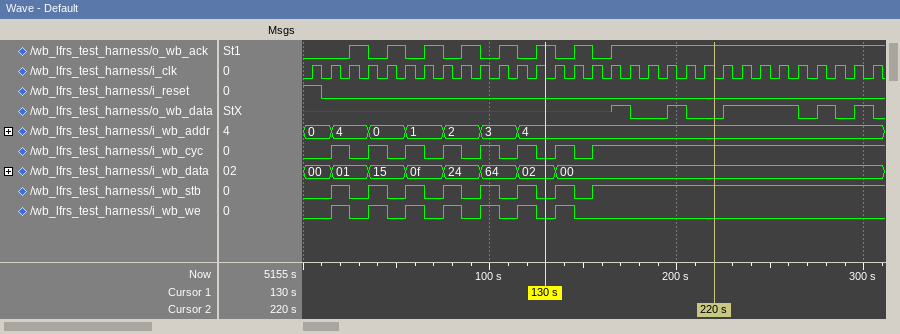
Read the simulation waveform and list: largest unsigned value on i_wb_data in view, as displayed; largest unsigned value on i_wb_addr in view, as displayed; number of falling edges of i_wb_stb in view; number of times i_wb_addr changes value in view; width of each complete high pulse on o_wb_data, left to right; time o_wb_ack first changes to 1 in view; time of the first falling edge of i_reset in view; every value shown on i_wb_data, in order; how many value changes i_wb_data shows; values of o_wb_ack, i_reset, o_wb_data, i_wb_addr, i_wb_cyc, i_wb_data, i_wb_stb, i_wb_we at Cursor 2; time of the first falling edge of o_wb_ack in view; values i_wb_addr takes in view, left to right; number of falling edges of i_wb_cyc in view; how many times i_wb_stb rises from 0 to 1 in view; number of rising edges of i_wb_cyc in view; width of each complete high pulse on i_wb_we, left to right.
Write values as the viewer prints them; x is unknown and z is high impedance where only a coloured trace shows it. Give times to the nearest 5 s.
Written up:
64
4
7
6
10 s, 40 s, 10 s, 10 s
25 s
10 s
00, 01, 15, 0f, 24, 64, 02, 00
7
o_wb_ack=1, i_reset=0, o_wb_data=0, i_wb_addr=4, i_wb_cyc=1, i_wb_data=00, i_wb_stb=1, i_wb_we=0
35 s
0, 4, 0, 1, 2, 3, 4
7
8
8
10 s, 10 s, 10 s, 10 s, 10 s, 10 s, 10 s
